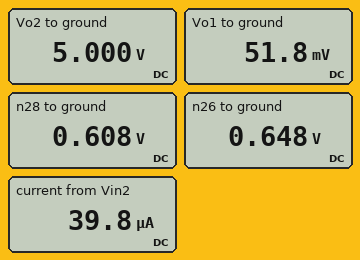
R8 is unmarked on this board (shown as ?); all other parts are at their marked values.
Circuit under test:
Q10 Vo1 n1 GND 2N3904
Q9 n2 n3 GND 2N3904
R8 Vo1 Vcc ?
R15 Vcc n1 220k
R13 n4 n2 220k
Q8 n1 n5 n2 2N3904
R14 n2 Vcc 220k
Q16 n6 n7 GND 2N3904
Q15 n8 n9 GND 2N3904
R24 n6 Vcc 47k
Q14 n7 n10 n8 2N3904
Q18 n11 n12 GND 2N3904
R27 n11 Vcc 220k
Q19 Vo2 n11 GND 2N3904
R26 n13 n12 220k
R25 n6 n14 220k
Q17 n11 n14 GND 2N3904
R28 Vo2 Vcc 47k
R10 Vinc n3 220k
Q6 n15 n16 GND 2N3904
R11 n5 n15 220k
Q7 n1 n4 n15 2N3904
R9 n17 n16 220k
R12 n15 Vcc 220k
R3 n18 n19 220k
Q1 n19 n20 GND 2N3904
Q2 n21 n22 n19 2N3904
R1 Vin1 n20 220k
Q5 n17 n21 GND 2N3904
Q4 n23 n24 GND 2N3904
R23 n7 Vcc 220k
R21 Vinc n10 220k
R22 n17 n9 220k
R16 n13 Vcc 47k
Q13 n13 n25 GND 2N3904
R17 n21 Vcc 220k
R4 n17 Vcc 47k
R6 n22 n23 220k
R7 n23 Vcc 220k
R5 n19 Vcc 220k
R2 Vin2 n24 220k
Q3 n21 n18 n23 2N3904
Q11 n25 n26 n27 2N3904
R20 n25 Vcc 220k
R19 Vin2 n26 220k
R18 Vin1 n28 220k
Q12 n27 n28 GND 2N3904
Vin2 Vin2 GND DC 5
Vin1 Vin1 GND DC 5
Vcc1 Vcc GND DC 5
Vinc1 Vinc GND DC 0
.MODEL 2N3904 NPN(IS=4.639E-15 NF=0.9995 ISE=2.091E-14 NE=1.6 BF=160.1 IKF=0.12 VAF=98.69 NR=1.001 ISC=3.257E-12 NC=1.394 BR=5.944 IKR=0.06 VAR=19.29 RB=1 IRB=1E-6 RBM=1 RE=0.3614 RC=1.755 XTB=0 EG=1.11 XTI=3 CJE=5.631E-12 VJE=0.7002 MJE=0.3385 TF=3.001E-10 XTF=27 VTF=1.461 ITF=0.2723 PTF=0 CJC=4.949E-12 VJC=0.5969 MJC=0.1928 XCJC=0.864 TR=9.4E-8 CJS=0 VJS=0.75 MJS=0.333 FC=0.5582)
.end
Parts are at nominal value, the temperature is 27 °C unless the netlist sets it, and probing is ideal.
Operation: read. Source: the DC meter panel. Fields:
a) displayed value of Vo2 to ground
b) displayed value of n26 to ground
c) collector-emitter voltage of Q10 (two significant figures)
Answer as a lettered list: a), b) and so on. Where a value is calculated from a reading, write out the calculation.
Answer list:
a) 5.000 V
b) 0.648 V
c) 51.8 mV = 52 mV
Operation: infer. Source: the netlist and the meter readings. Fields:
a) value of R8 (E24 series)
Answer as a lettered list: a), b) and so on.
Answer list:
a) 36 kΩ
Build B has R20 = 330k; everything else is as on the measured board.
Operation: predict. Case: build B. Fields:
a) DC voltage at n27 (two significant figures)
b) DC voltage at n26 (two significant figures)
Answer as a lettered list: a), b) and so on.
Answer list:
a) 46 mV
b) 640 mV
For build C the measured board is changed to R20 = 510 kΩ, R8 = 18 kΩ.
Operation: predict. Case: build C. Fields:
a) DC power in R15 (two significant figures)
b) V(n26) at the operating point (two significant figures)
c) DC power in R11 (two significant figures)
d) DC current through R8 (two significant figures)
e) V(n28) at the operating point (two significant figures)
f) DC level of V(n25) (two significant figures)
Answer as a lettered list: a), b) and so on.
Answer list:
a) 86 µW
b) 640 mV
c) 11 µW
d) 270 µA
e) 600 mV
f) 77 mV
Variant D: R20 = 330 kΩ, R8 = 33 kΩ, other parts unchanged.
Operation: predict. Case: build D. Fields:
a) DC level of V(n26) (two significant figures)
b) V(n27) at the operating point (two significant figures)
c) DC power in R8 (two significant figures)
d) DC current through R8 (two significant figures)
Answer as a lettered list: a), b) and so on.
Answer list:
a) 640 mV
b) 46 mV
c) 740 µW
d) 150 µA
